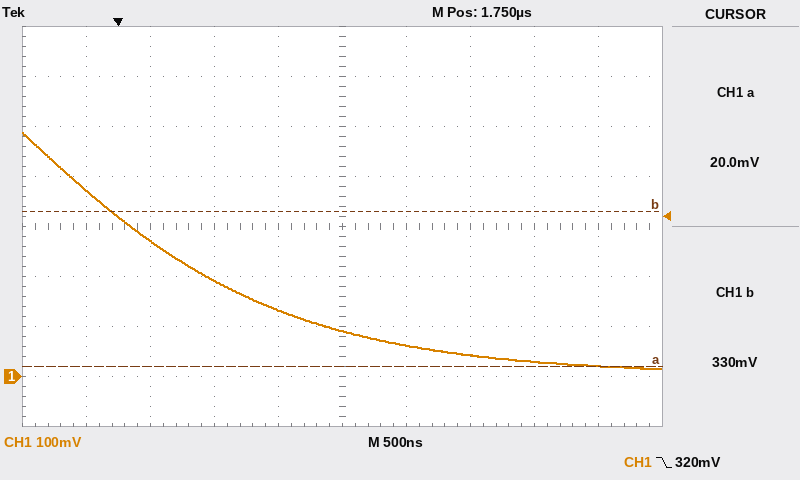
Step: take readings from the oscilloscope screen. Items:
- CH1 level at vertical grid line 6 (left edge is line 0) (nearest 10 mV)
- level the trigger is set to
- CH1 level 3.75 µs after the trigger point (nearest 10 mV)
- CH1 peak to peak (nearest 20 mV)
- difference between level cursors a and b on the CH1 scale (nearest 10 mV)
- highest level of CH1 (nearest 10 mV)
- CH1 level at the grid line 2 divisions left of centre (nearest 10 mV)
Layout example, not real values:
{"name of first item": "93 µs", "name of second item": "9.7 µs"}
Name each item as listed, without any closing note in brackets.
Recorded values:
{"CH1 level at vertical grid line 6 (left edge is line 0)": "60 mV", "level the trigger is set to": "320 mV", "CH1 level 3.75 µs after the trigger point": "20 mV", "CH1 peak to peak": "480 mV", "difference between level cursors a and b on the CH1 scale": "310 mV", "highest level of CH1": "490 mV", "CH1 level at the grid line 2 divisions left of centre": "190 mV"}
